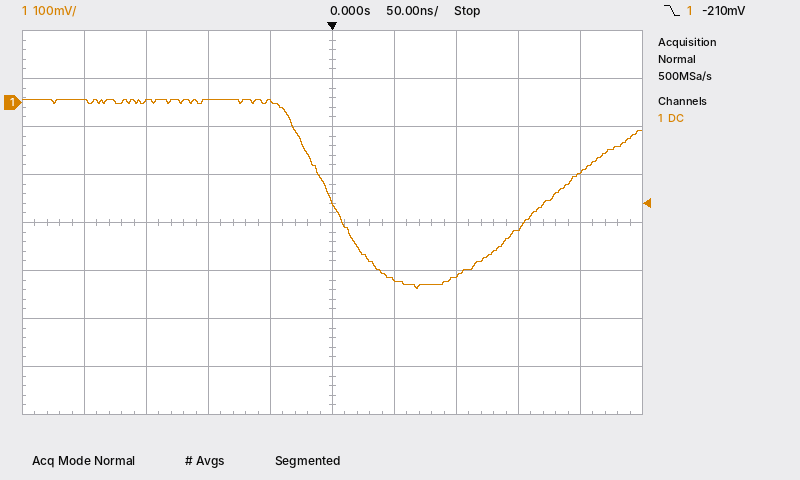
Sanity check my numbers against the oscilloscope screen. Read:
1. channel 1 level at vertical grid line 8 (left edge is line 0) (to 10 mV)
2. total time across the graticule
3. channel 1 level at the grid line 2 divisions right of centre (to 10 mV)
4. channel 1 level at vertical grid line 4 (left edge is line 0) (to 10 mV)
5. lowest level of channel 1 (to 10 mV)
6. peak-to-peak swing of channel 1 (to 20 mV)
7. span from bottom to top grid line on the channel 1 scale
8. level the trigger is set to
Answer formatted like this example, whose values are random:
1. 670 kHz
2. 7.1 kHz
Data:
1. -260 mV
2. 500 ns
3. -360 mV
4. 0 mV
5. -390 mV
6. 400 mV
7. 800 mV
8. -210 mV
